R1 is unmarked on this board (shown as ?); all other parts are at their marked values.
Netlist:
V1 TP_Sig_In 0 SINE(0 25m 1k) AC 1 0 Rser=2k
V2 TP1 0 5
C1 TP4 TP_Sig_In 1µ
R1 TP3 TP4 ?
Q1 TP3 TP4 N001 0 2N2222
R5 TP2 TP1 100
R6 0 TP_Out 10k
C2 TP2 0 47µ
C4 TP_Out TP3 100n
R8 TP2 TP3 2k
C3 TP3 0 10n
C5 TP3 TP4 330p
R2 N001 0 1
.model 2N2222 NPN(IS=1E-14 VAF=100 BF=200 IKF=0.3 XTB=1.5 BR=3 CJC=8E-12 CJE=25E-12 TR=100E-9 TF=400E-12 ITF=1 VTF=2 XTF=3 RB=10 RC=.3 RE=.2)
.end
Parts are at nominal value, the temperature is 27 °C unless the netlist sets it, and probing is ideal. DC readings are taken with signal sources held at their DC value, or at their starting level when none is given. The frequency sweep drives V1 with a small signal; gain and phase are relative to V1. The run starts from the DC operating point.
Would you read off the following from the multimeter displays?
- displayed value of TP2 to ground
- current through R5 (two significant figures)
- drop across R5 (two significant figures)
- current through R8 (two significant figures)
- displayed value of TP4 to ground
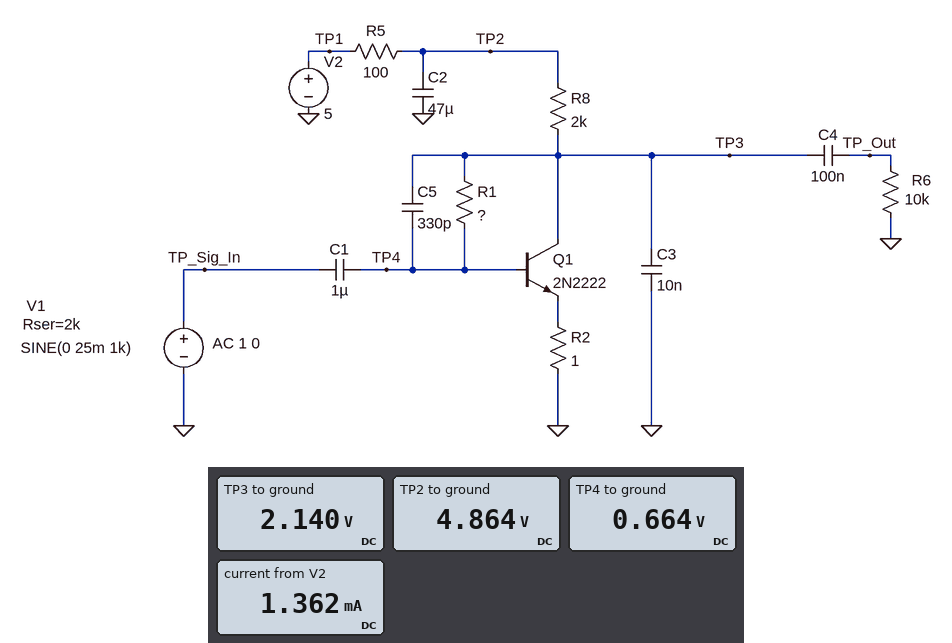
4.864 V
1.4 mA
140 mV
1.4 mA
0.664 V
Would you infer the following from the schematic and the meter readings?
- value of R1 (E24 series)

220 kΩ
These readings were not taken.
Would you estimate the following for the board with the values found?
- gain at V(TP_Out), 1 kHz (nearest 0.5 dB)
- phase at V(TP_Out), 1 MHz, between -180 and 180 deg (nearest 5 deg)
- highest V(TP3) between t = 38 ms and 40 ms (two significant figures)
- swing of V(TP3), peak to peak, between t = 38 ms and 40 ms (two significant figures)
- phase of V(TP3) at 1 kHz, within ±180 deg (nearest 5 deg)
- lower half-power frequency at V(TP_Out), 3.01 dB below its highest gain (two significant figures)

30.5 dB
40 deg
3.0 V
1.7 V
170 deg
140 Hz
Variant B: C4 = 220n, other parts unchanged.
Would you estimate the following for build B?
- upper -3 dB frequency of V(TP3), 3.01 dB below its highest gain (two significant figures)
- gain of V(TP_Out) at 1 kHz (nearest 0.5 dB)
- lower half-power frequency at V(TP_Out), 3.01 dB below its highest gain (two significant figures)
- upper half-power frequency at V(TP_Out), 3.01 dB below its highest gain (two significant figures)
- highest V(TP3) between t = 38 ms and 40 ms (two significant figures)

4.6 kHz
31.0 dB
81 Hz
4.7 kHz
3.0 V
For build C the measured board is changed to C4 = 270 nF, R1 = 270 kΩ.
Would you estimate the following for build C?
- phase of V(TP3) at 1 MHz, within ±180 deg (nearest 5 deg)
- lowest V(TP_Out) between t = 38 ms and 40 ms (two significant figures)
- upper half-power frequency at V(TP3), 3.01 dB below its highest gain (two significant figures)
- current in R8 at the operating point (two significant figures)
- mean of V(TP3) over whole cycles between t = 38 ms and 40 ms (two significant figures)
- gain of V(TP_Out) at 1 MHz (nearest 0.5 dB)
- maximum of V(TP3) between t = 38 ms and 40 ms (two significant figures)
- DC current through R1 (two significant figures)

40 deg
-910 mV
4.4 kHz
1.3 mA
2.3 V
-19.5 dB
3.2 V
6.2 µA
